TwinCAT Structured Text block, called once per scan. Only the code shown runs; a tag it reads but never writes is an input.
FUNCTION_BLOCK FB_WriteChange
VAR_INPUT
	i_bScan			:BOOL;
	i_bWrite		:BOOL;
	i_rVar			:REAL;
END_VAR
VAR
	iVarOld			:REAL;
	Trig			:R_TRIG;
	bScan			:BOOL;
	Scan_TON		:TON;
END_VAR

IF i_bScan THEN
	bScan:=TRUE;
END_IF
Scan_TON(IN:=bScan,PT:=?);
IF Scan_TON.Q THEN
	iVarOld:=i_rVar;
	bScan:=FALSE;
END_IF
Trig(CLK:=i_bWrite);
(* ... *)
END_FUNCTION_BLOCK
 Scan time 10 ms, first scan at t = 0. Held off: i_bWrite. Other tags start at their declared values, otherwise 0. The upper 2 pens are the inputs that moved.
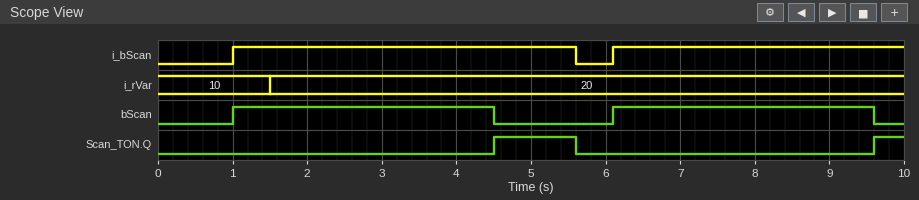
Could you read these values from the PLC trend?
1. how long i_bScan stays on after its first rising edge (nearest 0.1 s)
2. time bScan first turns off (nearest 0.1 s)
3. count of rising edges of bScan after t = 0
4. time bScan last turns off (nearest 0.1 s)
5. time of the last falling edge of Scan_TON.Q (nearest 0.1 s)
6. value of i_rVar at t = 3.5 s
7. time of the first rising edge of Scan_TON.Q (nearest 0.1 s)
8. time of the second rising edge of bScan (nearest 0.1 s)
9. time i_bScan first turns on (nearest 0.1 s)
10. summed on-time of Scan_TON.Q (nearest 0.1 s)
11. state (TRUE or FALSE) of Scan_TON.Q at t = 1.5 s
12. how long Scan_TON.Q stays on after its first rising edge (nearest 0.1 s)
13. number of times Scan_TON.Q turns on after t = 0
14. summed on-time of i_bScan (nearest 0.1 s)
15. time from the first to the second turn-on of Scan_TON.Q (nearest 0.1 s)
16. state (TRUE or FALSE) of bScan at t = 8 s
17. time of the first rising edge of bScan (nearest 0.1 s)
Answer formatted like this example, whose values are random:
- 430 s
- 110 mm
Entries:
- 4.6 s
- 4.5 s
- 2
- 9.6 s
- 5.6 s
- 20
- 4.5 s
- 6.1 s
- 1.0 s
- 1.5 s
- FALSE
- 1.1 s
- 2
- 8.5 s
- 5.1 s
- TRUE
- 1.0 s
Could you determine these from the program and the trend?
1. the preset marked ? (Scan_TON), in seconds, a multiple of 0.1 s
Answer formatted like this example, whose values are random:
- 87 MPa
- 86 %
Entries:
- 3.5 s
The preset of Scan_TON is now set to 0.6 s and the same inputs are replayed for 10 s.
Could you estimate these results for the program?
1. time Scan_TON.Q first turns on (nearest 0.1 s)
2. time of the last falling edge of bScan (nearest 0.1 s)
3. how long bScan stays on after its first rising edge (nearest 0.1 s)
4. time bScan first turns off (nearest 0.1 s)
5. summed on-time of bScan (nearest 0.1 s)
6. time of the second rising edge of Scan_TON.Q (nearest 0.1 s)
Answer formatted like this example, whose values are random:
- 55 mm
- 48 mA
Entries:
- 1.6 s
- 6.7 s
- 0.6 s
- 1.6 s
- 1.2 s
- 6.7 s
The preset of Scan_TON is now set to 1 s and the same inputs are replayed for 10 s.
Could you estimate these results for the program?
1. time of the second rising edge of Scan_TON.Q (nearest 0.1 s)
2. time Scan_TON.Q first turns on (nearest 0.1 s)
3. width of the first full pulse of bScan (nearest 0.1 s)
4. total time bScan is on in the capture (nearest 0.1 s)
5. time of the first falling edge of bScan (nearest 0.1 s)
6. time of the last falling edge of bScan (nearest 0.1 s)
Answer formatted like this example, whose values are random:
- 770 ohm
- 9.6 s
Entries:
- 7.1 s
- 2.0 s
- 1.0 s
- 2.0 s
- 2.0 s
- 7.1 s
